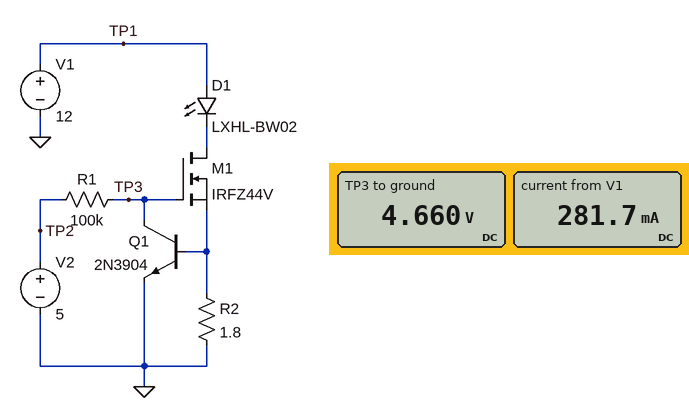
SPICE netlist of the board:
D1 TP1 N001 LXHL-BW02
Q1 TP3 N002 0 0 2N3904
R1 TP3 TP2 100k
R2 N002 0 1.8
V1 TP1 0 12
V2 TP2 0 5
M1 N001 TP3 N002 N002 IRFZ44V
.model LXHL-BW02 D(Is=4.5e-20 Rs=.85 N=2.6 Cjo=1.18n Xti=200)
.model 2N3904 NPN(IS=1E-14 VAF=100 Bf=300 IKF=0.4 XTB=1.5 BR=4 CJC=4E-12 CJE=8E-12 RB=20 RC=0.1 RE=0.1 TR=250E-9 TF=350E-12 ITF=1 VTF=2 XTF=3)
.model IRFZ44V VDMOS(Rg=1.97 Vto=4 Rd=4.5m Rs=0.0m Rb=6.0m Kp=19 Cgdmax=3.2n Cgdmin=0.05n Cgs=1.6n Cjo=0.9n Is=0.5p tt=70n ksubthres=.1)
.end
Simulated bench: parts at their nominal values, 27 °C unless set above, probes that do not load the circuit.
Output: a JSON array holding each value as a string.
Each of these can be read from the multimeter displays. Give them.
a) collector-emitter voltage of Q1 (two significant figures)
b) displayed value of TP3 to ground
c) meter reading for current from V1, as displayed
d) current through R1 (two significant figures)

["4.7 V", "4.660 V", "281.7 mA", "3.4 µA"]
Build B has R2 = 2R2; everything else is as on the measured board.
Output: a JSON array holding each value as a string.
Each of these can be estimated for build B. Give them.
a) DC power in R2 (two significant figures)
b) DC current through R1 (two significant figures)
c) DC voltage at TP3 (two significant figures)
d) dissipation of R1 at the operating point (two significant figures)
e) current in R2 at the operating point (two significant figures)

["120 mW", "3.6 µA", "4.6 V", "1.3 µW", "230 mA"]
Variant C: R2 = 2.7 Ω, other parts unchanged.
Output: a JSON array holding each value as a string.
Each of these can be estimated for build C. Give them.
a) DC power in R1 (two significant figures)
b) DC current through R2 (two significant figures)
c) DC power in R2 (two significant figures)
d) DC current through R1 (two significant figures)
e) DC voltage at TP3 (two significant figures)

["1.4 µW", "190 mA", "96 mW", "3.8 µA", "4.6 V"]
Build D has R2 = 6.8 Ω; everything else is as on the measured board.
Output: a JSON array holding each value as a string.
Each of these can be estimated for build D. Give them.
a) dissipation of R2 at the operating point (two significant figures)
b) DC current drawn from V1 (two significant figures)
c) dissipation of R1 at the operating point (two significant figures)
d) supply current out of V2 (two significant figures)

["39 mW", "76 mA", "2.0 µW", "4.5 µA"]
